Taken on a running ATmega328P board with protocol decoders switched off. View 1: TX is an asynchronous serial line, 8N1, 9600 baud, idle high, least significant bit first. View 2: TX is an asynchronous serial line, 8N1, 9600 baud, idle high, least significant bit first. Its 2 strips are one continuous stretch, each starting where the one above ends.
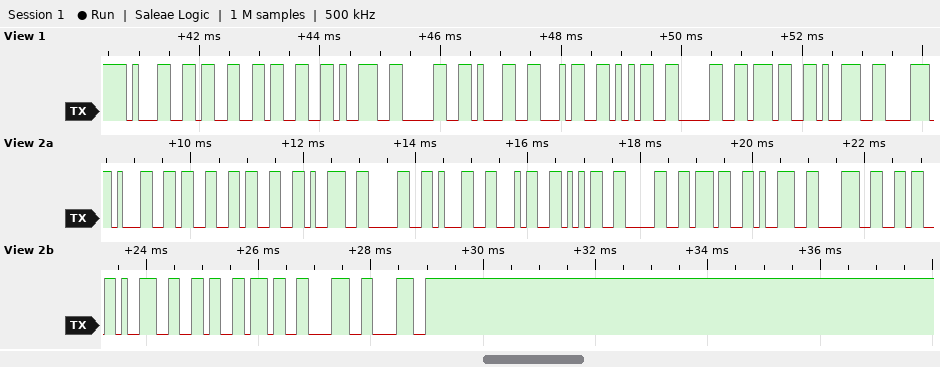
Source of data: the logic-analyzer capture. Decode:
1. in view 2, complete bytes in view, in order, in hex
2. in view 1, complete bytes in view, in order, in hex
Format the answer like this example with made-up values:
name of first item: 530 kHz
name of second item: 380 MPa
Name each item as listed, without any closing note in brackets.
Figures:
in view 2, complete bytes in view, in order, in hex: 0x31 0x33 0x33 0x39 0x30 0x31 0x34 0x35 0x30 0x37 0x39 0x38 0x36 0x39 0x36 0x37 0x38 0x38
in view 1, complete bytes in view, in order, in hex: 0x31 0x33 0x33 0x39 0x30 0x31 0x34 0x35 0x30 0x37 0x39
